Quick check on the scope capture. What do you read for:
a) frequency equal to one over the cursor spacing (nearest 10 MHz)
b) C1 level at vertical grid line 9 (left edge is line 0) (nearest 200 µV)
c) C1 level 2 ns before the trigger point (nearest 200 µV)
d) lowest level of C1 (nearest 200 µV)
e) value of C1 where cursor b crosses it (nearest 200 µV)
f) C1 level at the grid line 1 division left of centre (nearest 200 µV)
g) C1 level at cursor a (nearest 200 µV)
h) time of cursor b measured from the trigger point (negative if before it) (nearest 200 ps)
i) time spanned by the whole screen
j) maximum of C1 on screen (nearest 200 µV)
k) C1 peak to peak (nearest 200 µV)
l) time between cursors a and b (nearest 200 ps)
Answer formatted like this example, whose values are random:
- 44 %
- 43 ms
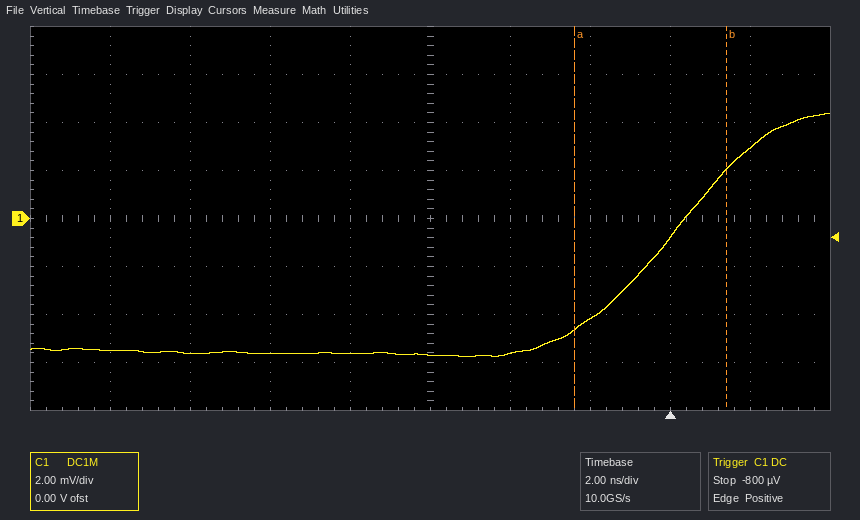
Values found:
- 260 MHz
- 3.0 mV
- -4.2 mV
- -5.8 mV
- 2.0 mV
- -5.6 mV
- -4.6 mV
- +1.4 ns
- 20 ns
- 4.4 mV
- 10.2 mV
- 3.8 ns
